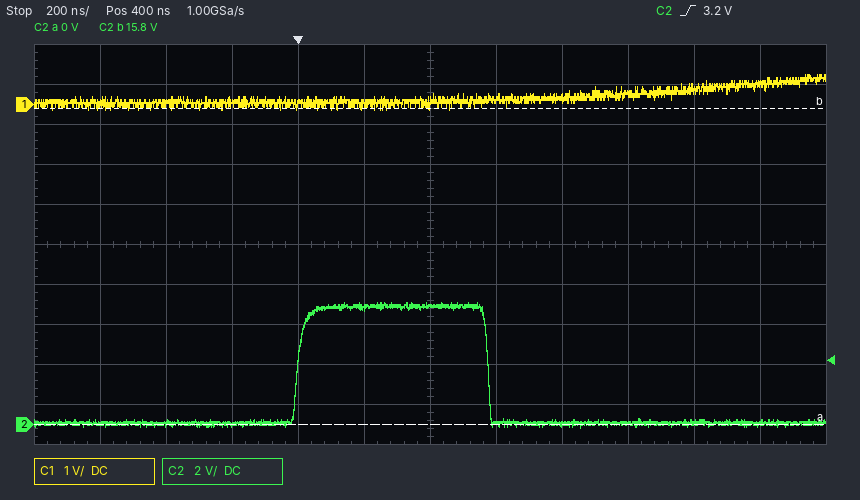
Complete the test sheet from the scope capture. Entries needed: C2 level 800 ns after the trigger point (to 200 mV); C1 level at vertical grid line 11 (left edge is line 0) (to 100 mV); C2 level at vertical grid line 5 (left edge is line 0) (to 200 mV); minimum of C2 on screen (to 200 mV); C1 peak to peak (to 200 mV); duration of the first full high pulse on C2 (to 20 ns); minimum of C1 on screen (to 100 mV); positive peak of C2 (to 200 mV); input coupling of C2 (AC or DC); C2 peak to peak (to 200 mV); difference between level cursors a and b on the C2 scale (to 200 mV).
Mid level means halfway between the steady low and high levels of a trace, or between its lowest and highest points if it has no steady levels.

0.0 V
500 mV
5.8 V
-200 mV
800 mV
580 ns
-100 mV
6.0 V
DC
6.2 V
15.8 V
